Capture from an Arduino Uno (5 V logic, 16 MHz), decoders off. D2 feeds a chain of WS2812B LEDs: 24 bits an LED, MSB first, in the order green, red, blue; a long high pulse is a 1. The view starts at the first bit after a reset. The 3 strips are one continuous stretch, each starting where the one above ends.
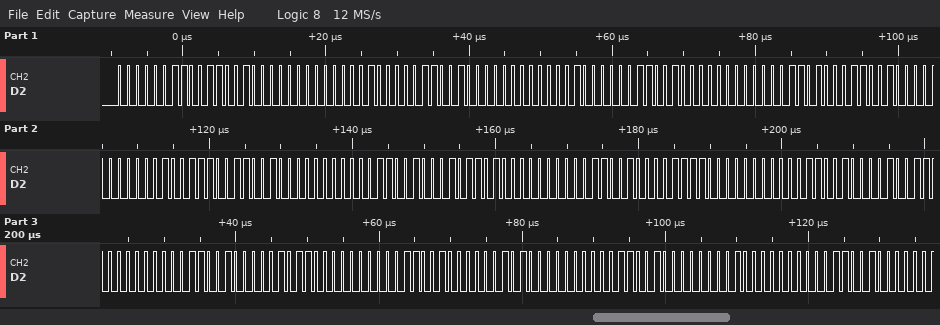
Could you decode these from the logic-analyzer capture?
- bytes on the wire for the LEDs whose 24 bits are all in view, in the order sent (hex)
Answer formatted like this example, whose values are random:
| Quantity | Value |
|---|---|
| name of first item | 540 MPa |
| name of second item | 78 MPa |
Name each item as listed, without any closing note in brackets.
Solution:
| Quantity | Value |
|---|---|
| bytes on the wire for the LEDs whose 24 bits are all in view, in the order sent | 03 32 00 08 32 00 10 32 00 1A 32 00 27 32 00 32 2D 00 32 1E 00 32 13 00 32 0B 00 32 05 00 32 01 00 |
